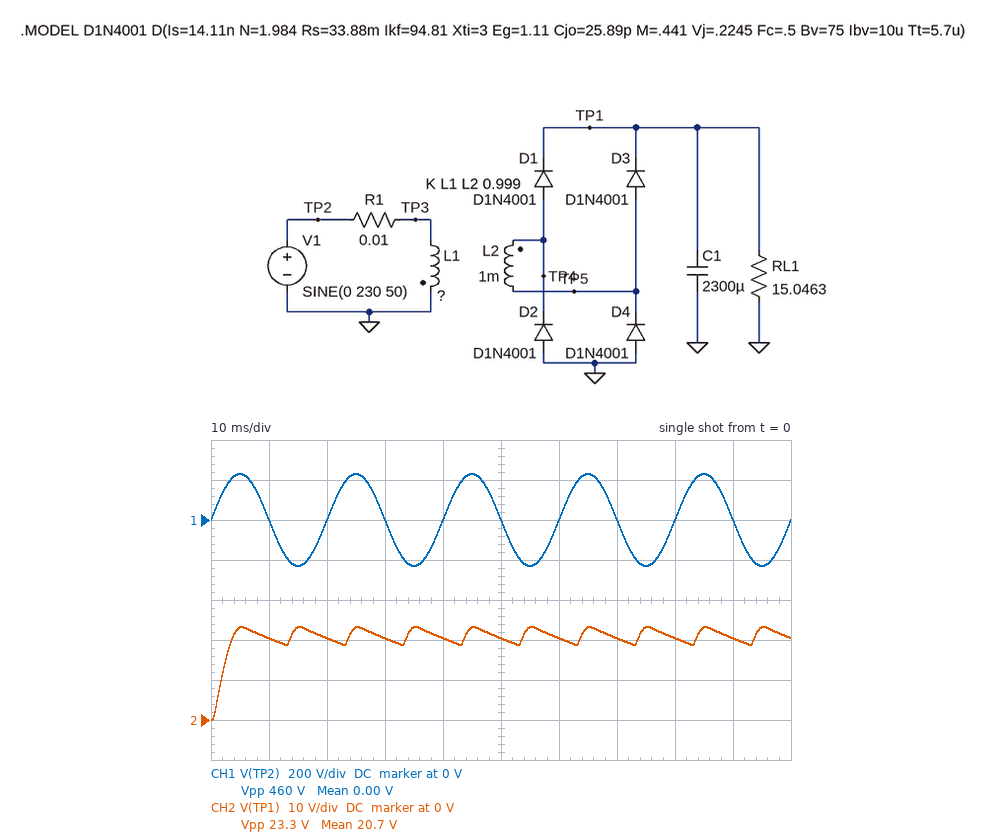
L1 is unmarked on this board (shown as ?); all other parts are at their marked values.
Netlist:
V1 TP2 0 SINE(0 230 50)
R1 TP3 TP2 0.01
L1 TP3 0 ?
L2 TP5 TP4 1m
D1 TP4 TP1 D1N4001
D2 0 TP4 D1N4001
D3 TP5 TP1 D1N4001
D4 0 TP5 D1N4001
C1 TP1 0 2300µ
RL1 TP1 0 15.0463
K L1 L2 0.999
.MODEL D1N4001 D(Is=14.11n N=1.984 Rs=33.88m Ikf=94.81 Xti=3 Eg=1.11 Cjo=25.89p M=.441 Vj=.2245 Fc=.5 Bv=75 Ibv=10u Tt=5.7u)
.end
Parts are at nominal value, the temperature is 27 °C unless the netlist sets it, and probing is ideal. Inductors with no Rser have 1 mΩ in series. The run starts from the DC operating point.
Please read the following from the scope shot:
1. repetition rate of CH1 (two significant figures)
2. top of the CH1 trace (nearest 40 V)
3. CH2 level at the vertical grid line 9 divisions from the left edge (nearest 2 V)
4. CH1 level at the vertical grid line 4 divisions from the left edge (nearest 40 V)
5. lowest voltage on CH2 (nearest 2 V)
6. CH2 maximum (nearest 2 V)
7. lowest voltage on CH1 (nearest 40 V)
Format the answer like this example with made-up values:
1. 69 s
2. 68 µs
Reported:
1. 50 Hz
2. 240 V
3. 20 V
4. 0 V
5. 0 V
6. 24 V
7. -240 V
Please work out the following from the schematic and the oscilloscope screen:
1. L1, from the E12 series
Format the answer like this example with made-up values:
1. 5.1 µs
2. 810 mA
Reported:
1. 82 mH
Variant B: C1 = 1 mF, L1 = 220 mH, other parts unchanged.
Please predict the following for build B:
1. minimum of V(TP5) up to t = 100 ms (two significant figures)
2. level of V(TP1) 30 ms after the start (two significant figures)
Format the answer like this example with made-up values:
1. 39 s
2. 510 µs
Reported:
1. -1.1 V
2. 10 V
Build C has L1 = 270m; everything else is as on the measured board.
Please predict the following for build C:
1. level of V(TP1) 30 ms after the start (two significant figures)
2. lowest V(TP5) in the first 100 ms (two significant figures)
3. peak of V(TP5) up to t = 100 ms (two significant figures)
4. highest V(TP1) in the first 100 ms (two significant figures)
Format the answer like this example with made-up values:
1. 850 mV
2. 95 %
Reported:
1. 11 V
2. -1.2 V
3. 13 V
4. 12 V
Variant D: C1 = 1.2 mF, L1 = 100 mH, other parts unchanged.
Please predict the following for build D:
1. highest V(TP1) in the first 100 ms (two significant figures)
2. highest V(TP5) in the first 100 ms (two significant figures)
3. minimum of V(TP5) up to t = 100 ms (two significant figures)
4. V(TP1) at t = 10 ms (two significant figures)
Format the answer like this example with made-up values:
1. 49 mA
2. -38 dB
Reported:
1. 21 V
2. 22 V
3. -1.3 V
4. 16 V
